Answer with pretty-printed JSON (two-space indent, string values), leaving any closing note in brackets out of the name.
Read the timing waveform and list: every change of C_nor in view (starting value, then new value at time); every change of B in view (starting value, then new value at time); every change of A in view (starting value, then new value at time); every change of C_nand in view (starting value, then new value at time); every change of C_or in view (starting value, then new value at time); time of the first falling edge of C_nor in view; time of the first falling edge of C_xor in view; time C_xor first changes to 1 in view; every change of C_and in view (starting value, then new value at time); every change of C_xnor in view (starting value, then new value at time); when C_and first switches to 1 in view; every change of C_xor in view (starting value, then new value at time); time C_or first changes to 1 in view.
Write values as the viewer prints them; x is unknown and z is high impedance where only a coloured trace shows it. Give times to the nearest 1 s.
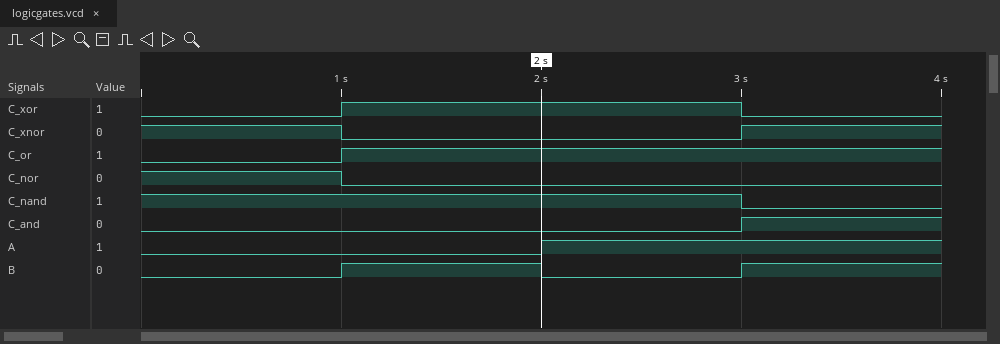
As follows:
{
  "every change of C_nor in view": "1, 0 at 1 s",
  "every change of B in view": "0, 1 at 1 s, 0 at 2 s, 1 at 3 s",
  "every change of A in view": "0, 1 at 2 s",
  "every change of C_nand in view": "1, 0 at 3 s",
  "every change of C_or in view": "0, 1 at 1 s",
  "time of the first falling edge of C_nor in view": "1 s",
  "time of the first falling edge of C_xor in view": "3 s",
  "time C_xor first changes to 1 in view": "1 s",
  "every change of C_and in view": "0, 1 at 3 s",
  "every change of C_xnor in view": "1, 0 at 1 s, 1 at 3 s",
  "when C_and first switches to 1 in view": "3 s",
  "every change of C_xor in view": "0, 1 at 1 s, 0 at 3 s",
  "time C_or first changes to 1 in view": "1 s"
}
